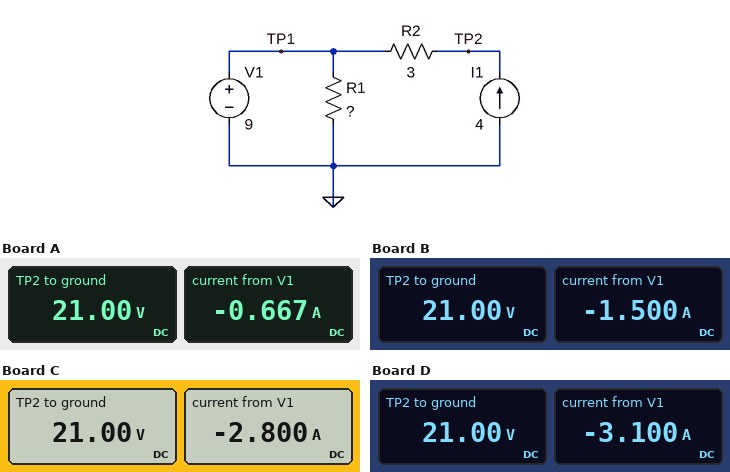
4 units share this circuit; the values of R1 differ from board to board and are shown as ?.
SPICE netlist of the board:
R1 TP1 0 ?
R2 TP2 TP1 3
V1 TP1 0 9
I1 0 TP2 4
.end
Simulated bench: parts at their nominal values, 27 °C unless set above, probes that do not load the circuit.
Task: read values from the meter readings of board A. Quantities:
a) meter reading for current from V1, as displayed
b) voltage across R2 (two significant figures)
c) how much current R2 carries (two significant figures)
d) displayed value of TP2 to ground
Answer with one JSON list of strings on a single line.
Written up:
["-0.667 A", "12 V", "4.0 A", "21.00 V"]
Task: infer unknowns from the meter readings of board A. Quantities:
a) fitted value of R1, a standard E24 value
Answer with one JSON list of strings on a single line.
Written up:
["2.7 Ω"]
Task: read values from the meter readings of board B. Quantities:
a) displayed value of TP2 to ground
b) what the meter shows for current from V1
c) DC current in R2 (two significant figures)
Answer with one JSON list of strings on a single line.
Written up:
["21.00 V", "-1.500 A", "4.0 A"]
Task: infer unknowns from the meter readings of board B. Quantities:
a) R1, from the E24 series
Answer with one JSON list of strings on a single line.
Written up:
["3.6 Ω"]
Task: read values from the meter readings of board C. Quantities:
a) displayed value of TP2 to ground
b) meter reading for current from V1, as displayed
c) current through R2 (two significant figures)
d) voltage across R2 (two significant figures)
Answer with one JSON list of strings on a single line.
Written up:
["21.00 V", "-2.800 A", "4.0 A", "12 V"]
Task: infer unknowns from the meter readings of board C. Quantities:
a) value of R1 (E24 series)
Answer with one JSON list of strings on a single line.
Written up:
["7.5 Ω"]
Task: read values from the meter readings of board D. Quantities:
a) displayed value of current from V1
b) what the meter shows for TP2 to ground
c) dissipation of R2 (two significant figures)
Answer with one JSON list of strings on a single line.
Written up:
["-3.100 A", "21.00 V", "48 W"]
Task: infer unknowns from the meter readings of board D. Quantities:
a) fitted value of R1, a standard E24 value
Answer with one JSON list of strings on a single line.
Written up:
["10 Ω"]
